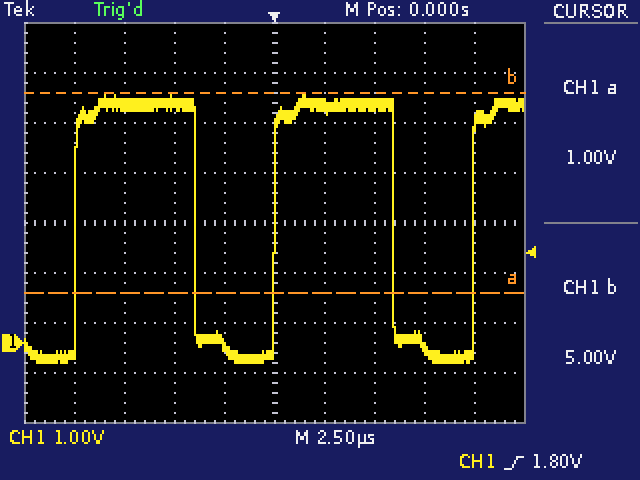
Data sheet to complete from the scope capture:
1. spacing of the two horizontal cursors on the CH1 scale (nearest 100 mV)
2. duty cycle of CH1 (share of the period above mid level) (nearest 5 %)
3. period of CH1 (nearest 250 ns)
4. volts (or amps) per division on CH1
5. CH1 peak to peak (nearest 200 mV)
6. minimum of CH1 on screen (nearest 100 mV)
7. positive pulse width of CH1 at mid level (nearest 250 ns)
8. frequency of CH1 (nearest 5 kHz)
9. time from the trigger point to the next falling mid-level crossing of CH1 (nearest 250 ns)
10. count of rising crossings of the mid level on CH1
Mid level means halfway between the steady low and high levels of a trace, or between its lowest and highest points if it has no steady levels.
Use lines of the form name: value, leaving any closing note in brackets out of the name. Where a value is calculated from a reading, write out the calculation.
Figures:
spacing of the two horizontal cursors on the CH1 scale: 4.0 V
duty cycle of CH1 (share of the period above mid level): 6.00 µs / 10.00 µs ≈ 60 %
period of CH1: 10.00 µs
volts (or amps) per division on CH1: 1 V
CH1 peak to peak: 5.4 V
minimum of CH1 on screen: -400 mV
positive pulse width of CH1 at mid level: 6.00 µs
frequency of CH1: 1 / 10.00 µs ≈ 100 kHz
time from the trigger point to the next falling mid-level crossing of CH1: 6.00 µs
count of rising crossings of the mid level on CH1: 3
